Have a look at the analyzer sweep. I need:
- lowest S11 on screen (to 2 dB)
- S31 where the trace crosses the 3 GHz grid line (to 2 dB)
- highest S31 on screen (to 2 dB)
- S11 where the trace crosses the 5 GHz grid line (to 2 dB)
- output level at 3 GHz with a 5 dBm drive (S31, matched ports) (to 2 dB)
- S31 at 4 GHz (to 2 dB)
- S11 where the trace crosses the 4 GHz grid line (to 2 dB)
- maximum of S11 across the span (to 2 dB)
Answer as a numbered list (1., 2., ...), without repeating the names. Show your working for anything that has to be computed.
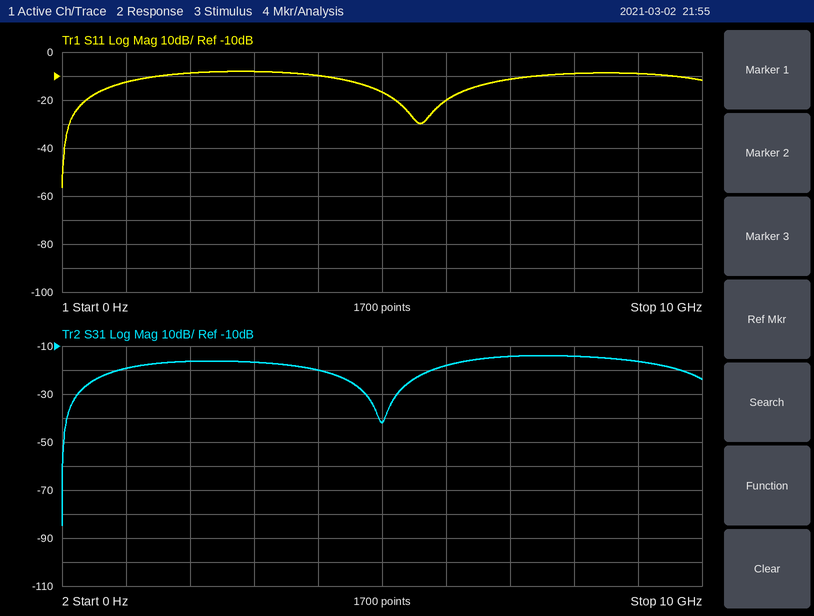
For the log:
1. -56 dB
2. -16 dB
3. -14 dB
4. -16 dB
5. 5 dBm + (-16 dB) = -12 dBm
6. -20 dB
7. -10 dB
8. -8 dB
